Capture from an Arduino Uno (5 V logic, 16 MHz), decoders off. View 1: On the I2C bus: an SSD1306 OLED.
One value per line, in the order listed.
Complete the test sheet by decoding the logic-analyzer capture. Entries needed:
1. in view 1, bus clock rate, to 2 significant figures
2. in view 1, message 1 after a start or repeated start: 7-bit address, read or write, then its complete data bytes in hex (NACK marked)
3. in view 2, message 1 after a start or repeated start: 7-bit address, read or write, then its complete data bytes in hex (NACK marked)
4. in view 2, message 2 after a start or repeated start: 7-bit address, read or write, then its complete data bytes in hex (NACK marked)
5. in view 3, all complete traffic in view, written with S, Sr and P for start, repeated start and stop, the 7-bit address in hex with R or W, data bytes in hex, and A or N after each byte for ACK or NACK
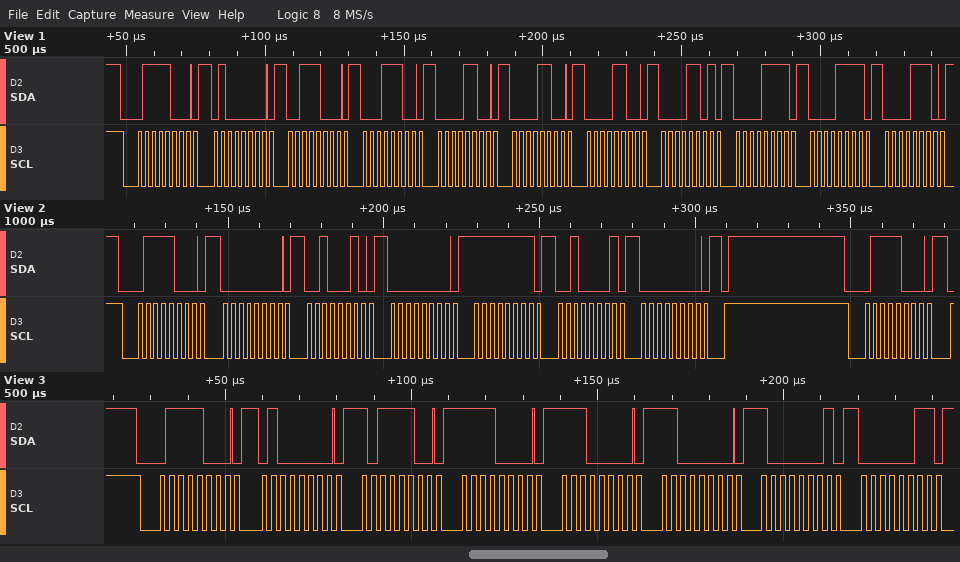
400 kHz
0x3C write: 40 38 1C 0C 0C 0C 0D 0F 0F 0E
0x3C write: 00 22 00 FF 21 00
0x3C write
S 3CW A 40 A BC A F0 A E0 A C0 A 81 A 03 A
